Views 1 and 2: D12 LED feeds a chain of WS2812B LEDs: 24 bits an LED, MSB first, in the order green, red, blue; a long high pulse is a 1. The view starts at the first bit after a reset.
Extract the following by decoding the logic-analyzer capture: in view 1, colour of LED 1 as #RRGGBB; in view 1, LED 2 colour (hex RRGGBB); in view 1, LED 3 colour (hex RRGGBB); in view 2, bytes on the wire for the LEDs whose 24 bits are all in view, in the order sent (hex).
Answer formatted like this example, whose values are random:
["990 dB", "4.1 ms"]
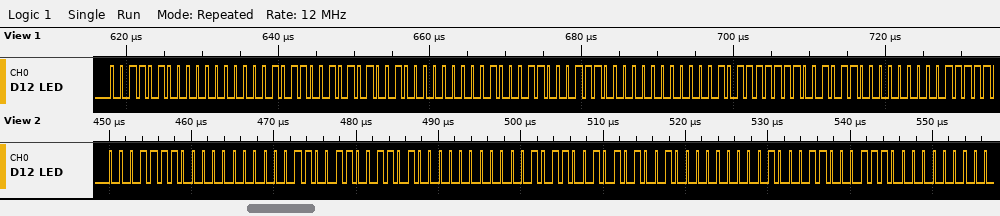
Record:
["#003459", "#00528C", "#0070BF", "1E 00 33 34 00 59 52 00 8C"]
